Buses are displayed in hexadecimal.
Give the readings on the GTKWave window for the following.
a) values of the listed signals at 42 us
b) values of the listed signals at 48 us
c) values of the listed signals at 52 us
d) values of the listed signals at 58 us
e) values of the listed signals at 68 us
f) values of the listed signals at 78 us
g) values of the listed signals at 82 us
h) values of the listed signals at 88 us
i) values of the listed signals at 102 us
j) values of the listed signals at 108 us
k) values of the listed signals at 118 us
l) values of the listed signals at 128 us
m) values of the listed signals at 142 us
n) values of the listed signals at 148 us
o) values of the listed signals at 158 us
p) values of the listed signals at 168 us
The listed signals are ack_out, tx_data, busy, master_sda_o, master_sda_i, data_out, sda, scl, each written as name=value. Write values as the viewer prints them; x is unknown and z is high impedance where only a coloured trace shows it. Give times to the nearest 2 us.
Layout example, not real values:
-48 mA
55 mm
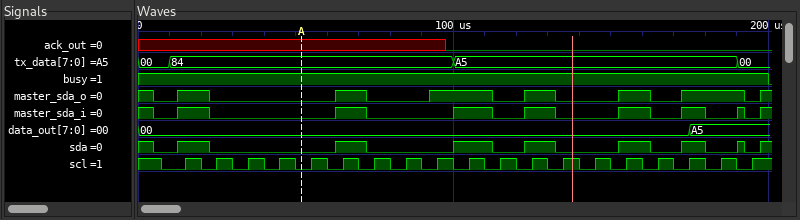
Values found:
ack_out=x, tx_data=84, busy=1, master_sda_o=0, master_sda_i=0, data_out=00, sda=0, scl=0
ack_out=x, tx_data=84, busy=1, master_sda_o=0, master_sda_i=0, data_out=00, sda=0, scl=1
ack_out=x, tx_data=84, busy=1, master_sda_o=0, master_sda_i=0, data_out=00, sda=0, scl=0
ack_out=x, tx_data=84, busy=1, master_sda_o=0, master_sda_i=0, data_out=00, sda=0, scl=1
ack_out=x, tx_data=84, busy=1, master_sda_o=1, master_sda_i=1, data_out=00, sda=1, scl=1
ack_out=x, tx_data=84, busy=1, master_sda_o=0, master_sda_i=0, data_out=00, sda=0, scl=1
ack_out=x, tx_data=84, busy=1, master_sda_o=0, master_sda_i=0, data_out=00, sda=0, scl=0
ack_out=x, tx_data=84, busy=1, master_sda_o=0, master_sda_i=0, data_out=00, sda=0, scl=1
ack_out=0, tx_data=A5, busy=1, master_sda_o=1, master_sda_i=1, data_out=00, sda=1, scl=0
ack_out=0, tx_data=A5, busy=1, master_sda_o=1, master_sda_i=1, data_out=00, sda=1, scl=1
ack_out=0, tx_data=A5, busy=1, master_sda_o=0, master_sda_i=0, data_out=00, sda=0, scl=1
ack_out=0, tx_data=A5, busy=1, master_sda_o=1, master_sda_i=1, data_out=00, sda=1, scl=1
ack_out=0, tx_data=A5, busy=1, master_sda_o=0, master_sda_i=0, data_out=00, sda=0, scl=0
ack_out=0, tx_data=A5, busy=1, master_sda_o=0, master_sda_i=0, data_out=00, sda=0, scl=1
ack_out=0, tx_data=A5, busy=1, master_sda_o=1, master_sda_i=1, data_out=00, sda=1, scl=1
ack_out=0, tx_data=A5, busy=1, master_sda_o=0, master_sda_i=0, data_out=00, sda=0, scl=1
